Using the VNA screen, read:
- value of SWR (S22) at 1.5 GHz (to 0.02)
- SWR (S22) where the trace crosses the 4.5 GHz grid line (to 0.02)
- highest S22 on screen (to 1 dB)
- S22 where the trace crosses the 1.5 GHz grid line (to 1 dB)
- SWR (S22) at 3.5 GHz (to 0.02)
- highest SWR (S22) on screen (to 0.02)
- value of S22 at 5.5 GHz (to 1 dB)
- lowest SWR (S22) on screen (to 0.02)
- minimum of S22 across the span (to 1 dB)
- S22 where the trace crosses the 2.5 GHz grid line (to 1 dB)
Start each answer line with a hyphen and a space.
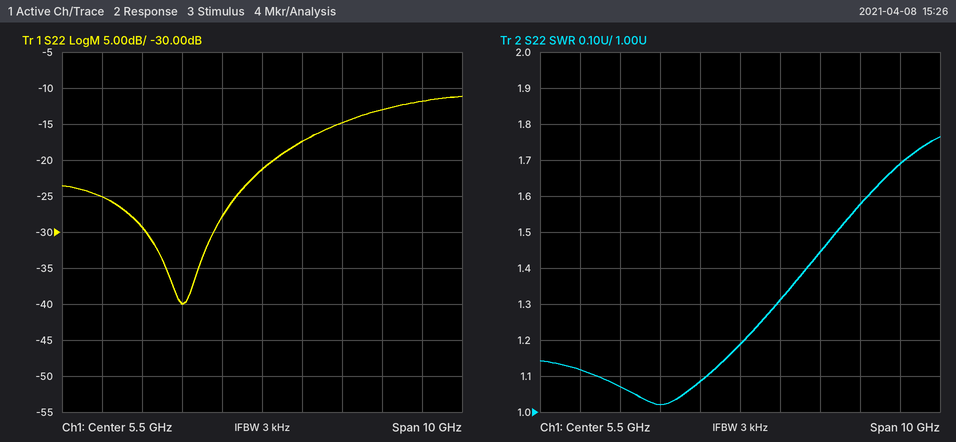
- 1.12
- 1.08
- -11 dB
- -25 dB
- 1.02
- 1.76
- -21 dB
- 1.02
- -40 dB
- -29 dB
